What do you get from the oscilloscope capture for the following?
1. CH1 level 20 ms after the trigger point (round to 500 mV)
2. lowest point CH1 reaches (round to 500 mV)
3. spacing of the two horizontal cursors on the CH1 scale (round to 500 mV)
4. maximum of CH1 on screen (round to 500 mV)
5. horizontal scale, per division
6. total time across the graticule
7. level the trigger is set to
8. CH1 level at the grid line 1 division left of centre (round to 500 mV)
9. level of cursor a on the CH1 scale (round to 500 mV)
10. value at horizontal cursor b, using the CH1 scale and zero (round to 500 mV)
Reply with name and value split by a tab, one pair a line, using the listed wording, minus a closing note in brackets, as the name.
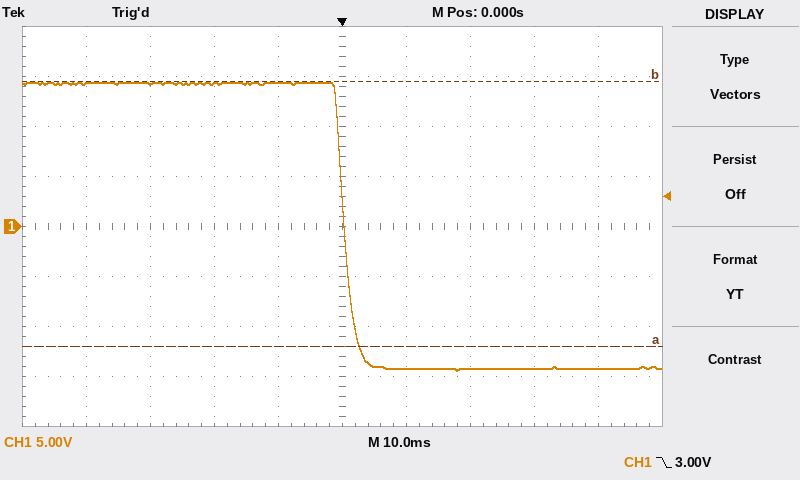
CH1 level 20 ms after the trigger point	-14.0 V
lowest point CH1 reaches	-14.5 V
spacing of the two horizontal cursors on the CH1 scale	26.5 V
maximum of CH1 on screen	14.5 V
horizontal scale, per division	10 ms
total time across the graticule	100 ms
level the trigger is set to	3.00 V
CH1 level at the grid line 1 division left of centre	14.5 V
level of cursor a on the CH1 scale	-12.0 V
value at horizontal cursor b, using the CH1 scale and zero	14.5 V
